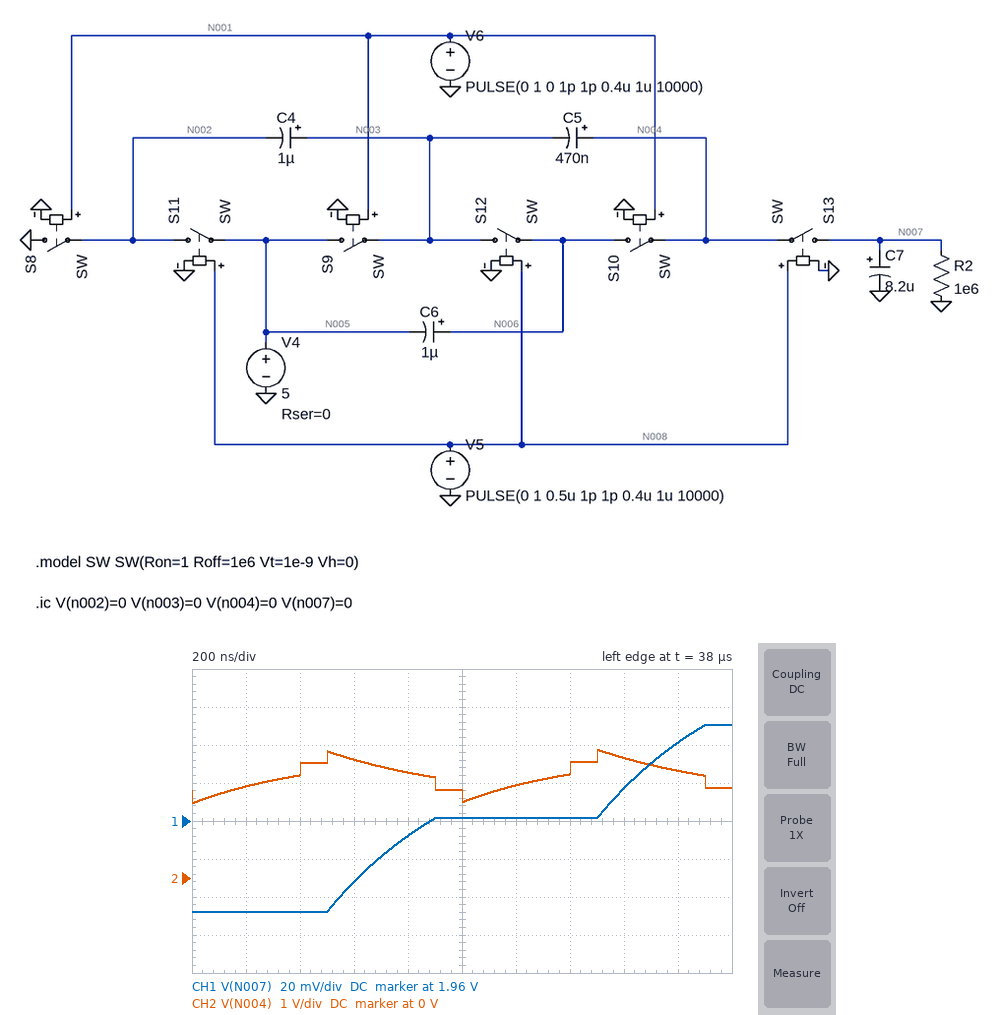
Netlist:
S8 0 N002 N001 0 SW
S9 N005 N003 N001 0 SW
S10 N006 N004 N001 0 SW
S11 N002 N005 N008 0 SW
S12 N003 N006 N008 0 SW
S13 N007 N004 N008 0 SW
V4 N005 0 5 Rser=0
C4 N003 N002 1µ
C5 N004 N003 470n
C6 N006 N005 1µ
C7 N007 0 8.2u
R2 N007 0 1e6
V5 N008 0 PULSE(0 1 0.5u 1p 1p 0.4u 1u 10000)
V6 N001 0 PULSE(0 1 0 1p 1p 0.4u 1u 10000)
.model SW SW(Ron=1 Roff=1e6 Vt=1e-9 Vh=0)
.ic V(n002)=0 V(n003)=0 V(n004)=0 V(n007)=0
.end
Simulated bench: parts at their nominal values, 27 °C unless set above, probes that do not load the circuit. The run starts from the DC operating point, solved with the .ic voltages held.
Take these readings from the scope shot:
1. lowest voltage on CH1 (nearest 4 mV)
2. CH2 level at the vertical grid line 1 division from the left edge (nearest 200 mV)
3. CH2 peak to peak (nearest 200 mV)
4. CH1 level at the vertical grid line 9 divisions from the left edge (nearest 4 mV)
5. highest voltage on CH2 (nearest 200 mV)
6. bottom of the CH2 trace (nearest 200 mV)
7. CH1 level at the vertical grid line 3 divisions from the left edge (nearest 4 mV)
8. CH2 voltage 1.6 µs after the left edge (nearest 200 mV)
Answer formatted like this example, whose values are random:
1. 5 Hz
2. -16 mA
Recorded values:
1. 1.912 V
2. 2.4 V
3. 1.4 V
4. 2.000 V
5. 3.4 V
6. 2.0 V
7. 1.928 V
8. 3.2 V
